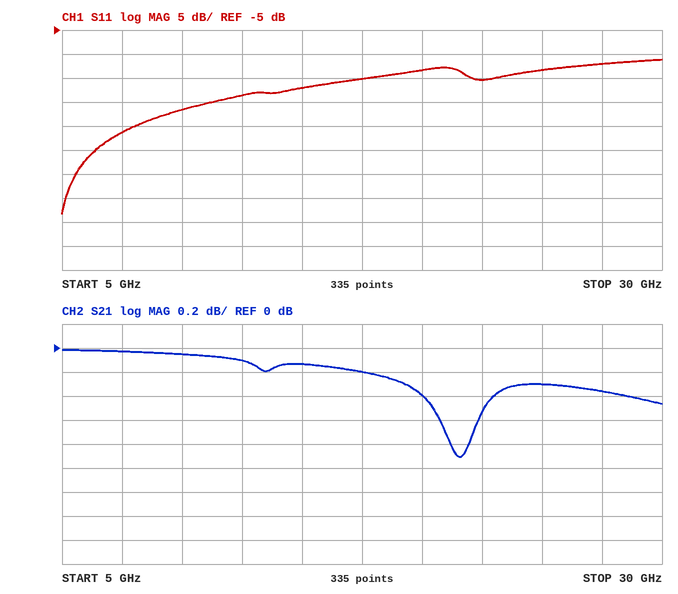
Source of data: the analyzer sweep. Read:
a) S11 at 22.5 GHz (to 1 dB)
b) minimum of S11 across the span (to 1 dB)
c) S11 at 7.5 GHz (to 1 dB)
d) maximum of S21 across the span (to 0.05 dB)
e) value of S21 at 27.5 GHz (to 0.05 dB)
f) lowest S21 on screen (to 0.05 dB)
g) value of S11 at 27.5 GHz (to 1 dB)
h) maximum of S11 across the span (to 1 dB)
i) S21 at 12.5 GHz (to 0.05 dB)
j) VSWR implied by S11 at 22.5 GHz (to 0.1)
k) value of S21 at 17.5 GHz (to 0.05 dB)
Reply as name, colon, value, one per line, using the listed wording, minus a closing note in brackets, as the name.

S11 at 22.5 GHz: -15 dB
minimum of S11 across the span: -43 dB
S11 at 7.5 GHz: -26 dB
maximum of S21 across the span: 0.00 dB
value of S21 at 27.5 GHz: -0.35 dB
lowest S21 on screen: -0.90 dB
value of S11 at 27.5 GHz: -12 dB
maximum of S11 across the span: -11 dB
S21 at 12.5 GHz: -0.10 dB
VSWR implied by S11 at 22.5 GHz: 1.4
value of S21 at 17.5 GHz: -0.20 dB
